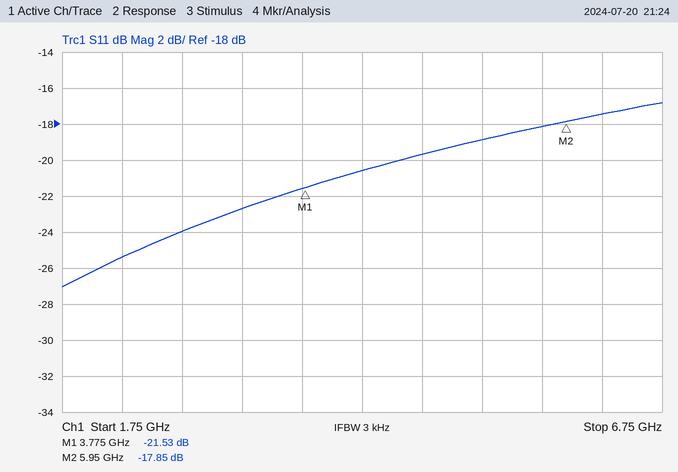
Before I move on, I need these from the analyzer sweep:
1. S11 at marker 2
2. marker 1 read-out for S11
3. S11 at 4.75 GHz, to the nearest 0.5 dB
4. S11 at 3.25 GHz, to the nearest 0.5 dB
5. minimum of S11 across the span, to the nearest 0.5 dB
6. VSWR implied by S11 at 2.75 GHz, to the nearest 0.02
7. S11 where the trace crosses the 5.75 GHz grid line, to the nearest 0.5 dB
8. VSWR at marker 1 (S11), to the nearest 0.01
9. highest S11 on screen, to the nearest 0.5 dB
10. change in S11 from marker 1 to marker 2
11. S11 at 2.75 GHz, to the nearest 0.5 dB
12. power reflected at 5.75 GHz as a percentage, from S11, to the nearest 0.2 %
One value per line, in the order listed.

-17.85 dB
-21.53 dB
-19.5 dB
-22.5 dB
-27.0 dB
1.14
-18.0 dB
1.18
-17.0 dB
3.68 dB
-24.0 dB
1.6 %
